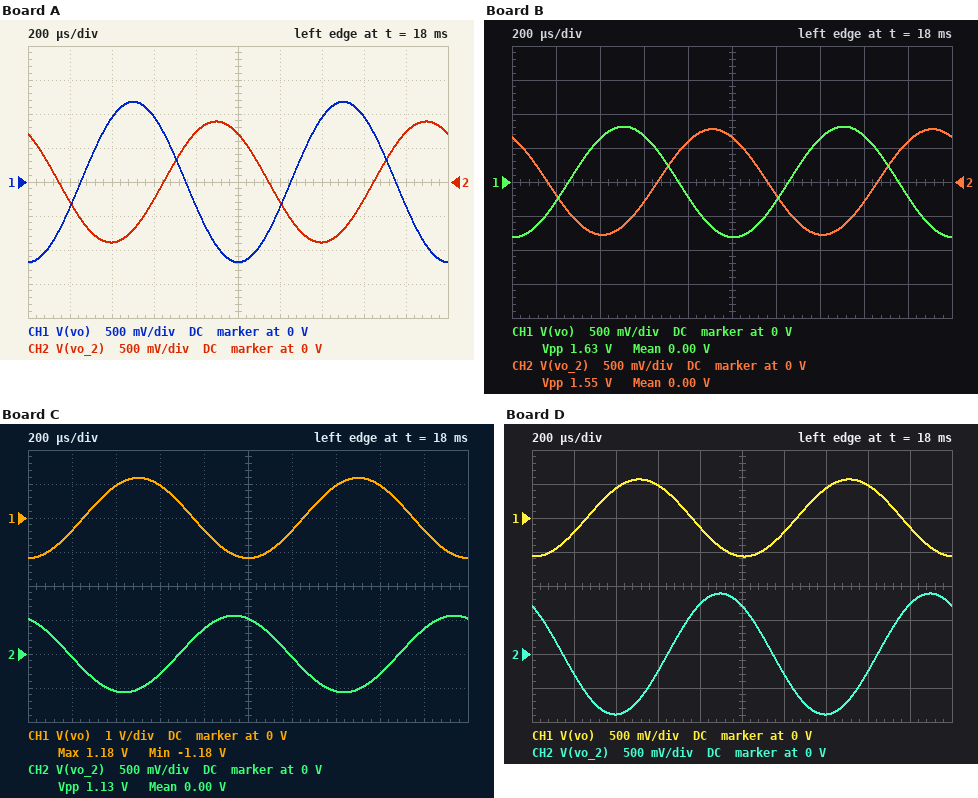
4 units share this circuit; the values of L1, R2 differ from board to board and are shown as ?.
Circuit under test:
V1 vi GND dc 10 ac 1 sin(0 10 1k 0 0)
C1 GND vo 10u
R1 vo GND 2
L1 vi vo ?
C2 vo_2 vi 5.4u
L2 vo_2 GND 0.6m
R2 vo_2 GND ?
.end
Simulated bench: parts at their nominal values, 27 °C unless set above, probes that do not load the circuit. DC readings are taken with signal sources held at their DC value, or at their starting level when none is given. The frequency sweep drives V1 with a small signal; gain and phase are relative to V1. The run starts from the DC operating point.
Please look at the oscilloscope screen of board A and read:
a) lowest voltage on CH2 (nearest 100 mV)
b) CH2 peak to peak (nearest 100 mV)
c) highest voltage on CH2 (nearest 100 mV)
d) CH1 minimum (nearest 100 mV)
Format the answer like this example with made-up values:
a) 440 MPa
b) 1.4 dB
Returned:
a) -900 mV
b) 1.8 V
c) 900 mV
d) -1.2 V
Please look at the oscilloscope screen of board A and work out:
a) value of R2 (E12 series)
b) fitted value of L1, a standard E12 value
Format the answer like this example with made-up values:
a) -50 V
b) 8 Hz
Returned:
a) 3.3 Ω
b) 2.7 mH
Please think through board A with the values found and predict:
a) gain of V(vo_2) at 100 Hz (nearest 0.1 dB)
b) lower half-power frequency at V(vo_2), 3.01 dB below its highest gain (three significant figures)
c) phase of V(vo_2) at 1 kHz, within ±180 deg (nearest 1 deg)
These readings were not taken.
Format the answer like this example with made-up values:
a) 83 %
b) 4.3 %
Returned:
a) -57.9 dB
b) 8.07 kHz
c) 127 deg
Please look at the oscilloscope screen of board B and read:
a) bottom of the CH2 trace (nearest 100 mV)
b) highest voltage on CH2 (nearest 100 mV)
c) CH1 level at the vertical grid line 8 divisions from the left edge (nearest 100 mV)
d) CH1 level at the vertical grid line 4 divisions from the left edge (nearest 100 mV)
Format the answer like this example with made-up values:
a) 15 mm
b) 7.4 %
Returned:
a) -800 mV
b) 800 mV
c) 700 mV
d) -200 mV
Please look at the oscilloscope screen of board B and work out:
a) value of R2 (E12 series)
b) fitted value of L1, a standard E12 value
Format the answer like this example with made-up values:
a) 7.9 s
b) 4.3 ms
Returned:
a) 2.7 Ω
b) 3.9 mH
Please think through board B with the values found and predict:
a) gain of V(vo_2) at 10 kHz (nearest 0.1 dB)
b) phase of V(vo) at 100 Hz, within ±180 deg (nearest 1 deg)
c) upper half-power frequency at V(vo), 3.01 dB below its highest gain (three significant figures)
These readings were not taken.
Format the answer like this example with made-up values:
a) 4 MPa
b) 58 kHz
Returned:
a) -3.1 dB
b) -51 deg
c) 82.5 Hz
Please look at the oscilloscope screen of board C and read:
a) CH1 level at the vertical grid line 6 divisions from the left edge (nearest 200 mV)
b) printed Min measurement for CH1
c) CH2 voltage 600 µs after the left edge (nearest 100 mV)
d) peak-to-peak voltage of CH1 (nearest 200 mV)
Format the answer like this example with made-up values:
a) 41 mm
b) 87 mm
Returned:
a) -400 mV
b) -1.18 V
c) -300 mV
d) 2.4 V
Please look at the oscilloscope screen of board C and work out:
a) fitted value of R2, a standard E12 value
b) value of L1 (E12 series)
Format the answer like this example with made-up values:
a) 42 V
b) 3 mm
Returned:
a) 1.8 Ω
b) 2.7 mH
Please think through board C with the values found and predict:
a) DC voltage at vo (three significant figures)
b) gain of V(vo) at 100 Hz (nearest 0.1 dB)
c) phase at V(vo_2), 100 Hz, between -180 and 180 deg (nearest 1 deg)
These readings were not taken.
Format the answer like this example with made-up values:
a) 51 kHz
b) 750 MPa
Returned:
a) 10.0 V
b) -2.3 dB
c) 168 deg
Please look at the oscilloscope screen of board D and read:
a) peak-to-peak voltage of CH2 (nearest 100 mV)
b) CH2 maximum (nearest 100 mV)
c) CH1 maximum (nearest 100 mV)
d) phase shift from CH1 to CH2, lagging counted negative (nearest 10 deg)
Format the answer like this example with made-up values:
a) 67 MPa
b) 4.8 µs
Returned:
a) 1.8 V
b) 900 mV
c) 600 mV
d) -140 deg
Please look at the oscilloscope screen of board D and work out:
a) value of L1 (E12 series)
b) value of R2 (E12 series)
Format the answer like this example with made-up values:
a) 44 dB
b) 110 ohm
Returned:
a) 5.6 mH
b) 3.3 Ω
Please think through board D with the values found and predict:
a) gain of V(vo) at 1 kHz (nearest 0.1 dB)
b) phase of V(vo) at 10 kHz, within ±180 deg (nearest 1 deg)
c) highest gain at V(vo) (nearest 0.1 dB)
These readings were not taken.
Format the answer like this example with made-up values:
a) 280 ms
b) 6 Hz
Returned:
a) -24.9 dB
b) -141 deg
c) 0 dB
